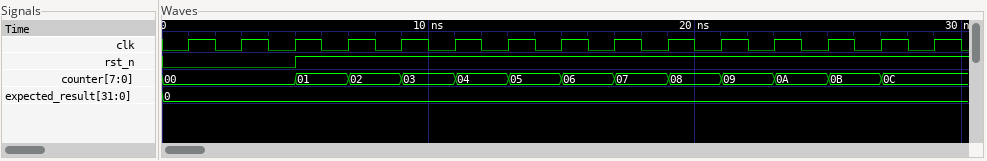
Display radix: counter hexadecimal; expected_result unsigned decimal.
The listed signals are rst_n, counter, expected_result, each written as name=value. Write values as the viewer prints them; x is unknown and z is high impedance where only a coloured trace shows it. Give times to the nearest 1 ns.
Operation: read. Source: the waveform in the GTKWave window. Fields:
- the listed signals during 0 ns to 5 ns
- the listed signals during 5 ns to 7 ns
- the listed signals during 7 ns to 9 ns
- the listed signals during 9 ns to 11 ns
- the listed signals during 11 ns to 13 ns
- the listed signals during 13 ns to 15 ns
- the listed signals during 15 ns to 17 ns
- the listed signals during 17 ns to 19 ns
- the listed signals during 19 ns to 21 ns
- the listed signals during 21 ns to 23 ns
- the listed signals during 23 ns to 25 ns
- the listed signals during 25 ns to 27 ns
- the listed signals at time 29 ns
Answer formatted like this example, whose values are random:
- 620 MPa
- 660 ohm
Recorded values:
- rst_n=0, counter=00, expected_result=0
- rst_n=1, counter=01, expected_result=0
- rst_n=1, counter=02, expected_result=0
- rst_n=1, counter=03, expected_result=0
- rst_n=1, counter=04, expected_result=0
- rst_n=1, counter=05, expected_result=0
- rst_n=1, counter=06, expected_result=0
- rst_n=1, counter=07, expected_result=0
- rst_n=1, counter=08, expected_result=0
- rst_n=1, counter=09, expected_result=0
- rst_n=1, counter=0A, expected_result=0
- rst_n=1, counter=0B, expected_result=0
- rst_n=1, counter=0C, expected_result=0
